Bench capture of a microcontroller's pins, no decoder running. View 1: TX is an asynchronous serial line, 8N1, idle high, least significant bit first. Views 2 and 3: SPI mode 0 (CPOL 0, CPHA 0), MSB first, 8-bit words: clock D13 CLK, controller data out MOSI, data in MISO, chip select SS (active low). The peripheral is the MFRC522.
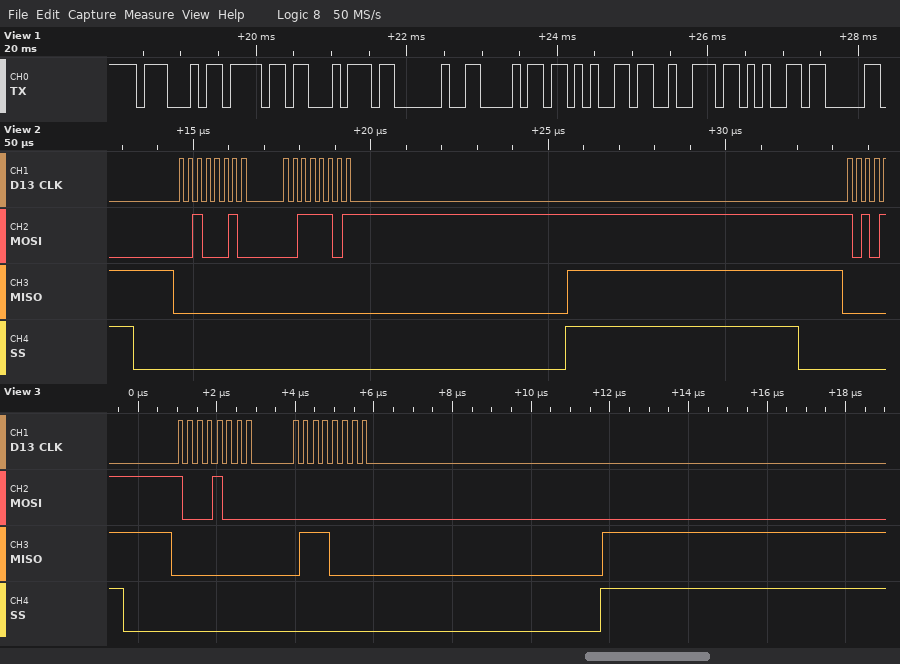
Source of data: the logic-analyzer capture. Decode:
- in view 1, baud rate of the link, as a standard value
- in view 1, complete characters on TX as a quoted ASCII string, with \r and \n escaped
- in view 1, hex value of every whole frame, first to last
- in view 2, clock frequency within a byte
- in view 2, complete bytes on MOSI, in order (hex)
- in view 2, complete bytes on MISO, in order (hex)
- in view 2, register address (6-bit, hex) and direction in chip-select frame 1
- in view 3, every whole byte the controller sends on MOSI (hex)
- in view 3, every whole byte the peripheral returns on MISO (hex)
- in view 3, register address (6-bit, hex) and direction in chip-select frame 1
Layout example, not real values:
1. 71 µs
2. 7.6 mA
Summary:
1. 9600 baud
2. "Got here"
3. 47 6F 74 20 68 65 72 65
4. 4 MHz
5. 22 3D
6. 00 00
7. 0x11 write
8. 88 00
9. 00 70
10. 0x04 read
